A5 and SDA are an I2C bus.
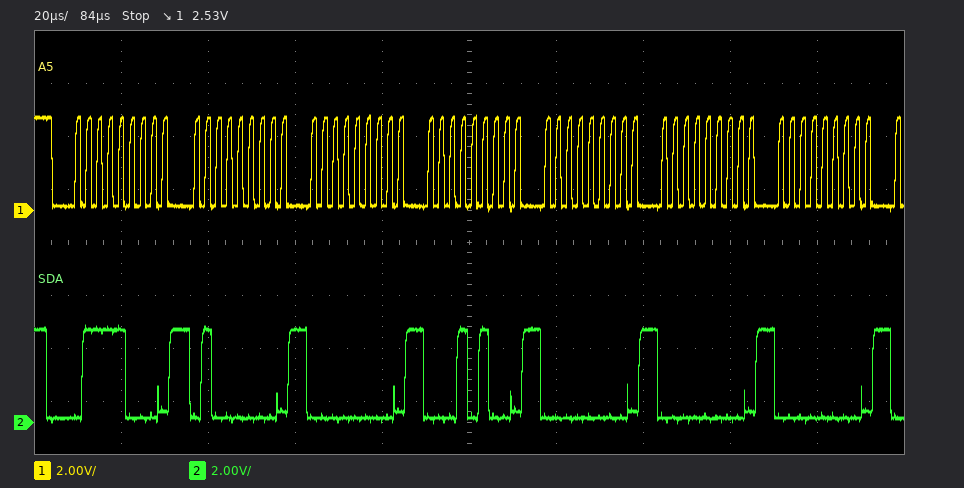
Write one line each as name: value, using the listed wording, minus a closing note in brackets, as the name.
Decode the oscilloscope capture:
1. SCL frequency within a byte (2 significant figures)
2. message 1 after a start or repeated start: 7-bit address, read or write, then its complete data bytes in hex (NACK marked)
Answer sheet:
SCL frequency within a byte: 400 kHz
message 1 after a start or repeated start: 7-bit address, read or write, then its complete data bytes in hex: 0x3C write: 40 00 14 00 00 00
